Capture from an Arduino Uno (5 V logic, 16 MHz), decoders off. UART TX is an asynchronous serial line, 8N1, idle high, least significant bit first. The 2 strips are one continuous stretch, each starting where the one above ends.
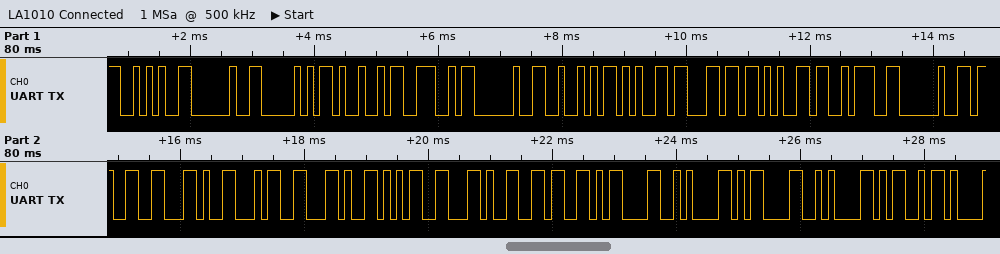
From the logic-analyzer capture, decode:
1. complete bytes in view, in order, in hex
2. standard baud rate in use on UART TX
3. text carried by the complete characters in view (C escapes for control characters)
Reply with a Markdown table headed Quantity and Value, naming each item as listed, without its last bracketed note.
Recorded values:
| Quantity | Value |
|---|---|
| complete bytes in view, in order, in hex | 0x2A 0x20 0x50 0x49 0x4E 0x20 0x52 0x65 0x6C 0x65 0x3A 0x20 0x33 0x2C 0x34 0x2C 0x35 0x2C 0x36 0x0D 0x0A 0x0D 0x0A 0x4D |
| standard baud rate in use on UART TX | 9600 baud |
| text carried by the complete characters in view | "* PIN Rele: 3,4,5,6\r\n\r\nM" |
